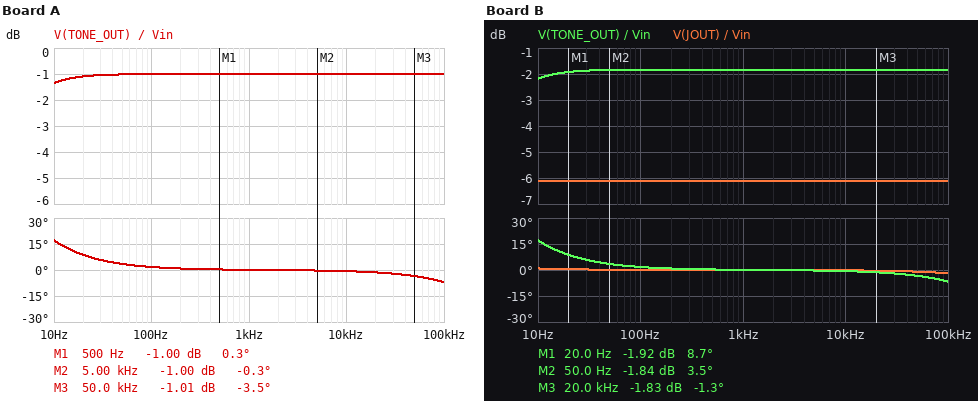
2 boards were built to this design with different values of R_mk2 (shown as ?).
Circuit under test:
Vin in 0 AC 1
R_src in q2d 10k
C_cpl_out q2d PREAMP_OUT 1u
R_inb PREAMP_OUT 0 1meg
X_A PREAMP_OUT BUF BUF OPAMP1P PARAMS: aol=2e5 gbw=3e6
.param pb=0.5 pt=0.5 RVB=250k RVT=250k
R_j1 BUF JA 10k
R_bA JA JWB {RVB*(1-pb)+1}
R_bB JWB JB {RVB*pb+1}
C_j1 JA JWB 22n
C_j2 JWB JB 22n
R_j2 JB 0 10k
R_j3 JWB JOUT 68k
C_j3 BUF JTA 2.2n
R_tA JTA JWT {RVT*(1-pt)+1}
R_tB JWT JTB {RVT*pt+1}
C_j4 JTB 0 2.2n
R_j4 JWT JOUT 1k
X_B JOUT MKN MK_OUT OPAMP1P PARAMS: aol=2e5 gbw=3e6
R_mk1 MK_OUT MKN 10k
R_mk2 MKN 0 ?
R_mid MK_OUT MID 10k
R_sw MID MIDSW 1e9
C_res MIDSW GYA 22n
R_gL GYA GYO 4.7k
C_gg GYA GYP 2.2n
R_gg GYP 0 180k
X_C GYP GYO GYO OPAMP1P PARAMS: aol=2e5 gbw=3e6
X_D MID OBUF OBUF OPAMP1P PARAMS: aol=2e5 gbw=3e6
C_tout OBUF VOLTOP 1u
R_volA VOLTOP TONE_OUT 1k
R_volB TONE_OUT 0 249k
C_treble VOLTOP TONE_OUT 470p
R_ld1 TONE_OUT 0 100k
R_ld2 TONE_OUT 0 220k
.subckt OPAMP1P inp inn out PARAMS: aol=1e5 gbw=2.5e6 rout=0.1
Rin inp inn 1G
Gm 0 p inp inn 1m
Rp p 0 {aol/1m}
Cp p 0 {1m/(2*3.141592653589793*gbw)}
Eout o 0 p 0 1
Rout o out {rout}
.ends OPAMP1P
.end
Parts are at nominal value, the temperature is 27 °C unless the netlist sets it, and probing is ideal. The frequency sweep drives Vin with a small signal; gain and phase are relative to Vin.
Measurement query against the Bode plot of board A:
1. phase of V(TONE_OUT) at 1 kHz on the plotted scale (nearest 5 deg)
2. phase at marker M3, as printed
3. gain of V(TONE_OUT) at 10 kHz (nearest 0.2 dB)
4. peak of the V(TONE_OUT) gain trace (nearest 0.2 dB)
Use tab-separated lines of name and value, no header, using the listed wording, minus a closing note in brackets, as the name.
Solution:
phase of V(TONE_OUT) at 1 kHz on the plotted scale	0 deg
phase at marker M3, as printed	-3.5 deg
gain of V(TONE_OUT) at 10 kHz	-1.0 dB
peak of the V(TONE_OUT) gain trace	-1.0 dB
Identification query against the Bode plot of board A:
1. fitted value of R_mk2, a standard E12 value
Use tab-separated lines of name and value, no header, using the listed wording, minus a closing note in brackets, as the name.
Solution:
fitted value of R_mk2, a standard E12 value	12 kΩ
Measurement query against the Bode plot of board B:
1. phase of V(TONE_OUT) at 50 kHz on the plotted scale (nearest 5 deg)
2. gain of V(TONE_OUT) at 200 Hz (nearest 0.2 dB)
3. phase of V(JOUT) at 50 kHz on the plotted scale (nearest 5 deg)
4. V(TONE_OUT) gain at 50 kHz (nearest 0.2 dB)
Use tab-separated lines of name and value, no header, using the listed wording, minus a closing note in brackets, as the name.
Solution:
phase of V(TONE_OUT) at 50 kHz on the plotted scale	-5 deg
gain of V(TONE_OUT) at 200 Hz	-1.8 dB
phase of V(JOUT) at 50 kHz on the plotted scale	0 deg
V(TONE_OUT) gain at 50 kHz	-1.8 dB
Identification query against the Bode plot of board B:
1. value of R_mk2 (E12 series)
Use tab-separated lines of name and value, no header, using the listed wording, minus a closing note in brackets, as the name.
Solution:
value of R_mk2	15 kΩ
